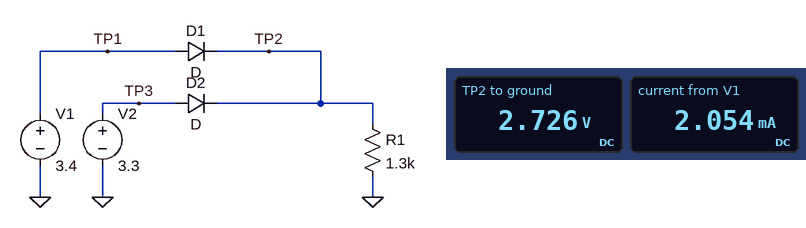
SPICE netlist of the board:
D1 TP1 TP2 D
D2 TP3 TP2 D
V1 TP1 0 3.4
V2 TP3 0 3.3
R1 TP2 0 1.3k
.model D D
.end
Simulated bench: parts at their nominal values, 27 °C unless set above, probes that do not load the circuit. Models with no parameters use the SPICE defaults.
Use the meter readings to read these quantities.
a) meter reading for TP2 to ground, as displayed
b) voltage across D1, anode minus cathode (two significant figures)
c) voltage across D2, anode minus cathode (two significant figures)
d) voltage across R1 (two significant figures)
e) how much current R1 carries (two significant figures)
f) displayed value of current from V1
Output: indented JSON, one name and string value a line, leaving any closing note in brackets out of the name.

{
  "meter reading for TP2 to ground, as displayed": "2.726 V",
  "voltage across D1, anode minus cathode": "670 mV",
  "voltage across D2, anode minus cathode": "570 mV",
  "voltage across R1": "2.7 V",
  "how much current R1 carries": "2.1 mA",
  "displayed value of current from V1": "2.054 mA"
}
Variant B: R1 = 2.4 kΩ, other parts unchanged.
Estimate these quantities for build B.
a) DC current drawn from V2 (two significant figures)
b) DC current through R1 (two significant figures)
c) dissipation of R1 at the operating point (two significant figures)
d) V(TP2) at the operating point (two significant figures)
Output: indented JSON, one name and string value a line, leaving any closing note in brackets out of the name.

{
  "DC current drawn from V2": "23 µA",
  "DC current through R1": "1.1 mA",
  "dissipation of R1 at the operating point": "3.1 mW",
  "V(TP2) at the operating point": "2.7 V"
}
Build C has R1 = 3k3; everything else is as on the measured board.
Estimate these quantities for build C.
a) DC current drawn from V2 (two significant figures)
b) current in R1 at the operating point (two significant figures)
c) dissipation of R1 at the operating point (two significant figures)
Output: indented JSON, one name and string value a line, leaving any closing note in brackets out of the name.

{
  "DC current drawn from V2": "17 µA",
  "current in R1 at the operating point": "830 µA",
  "dissipation of R1 at the operating point": "2.3 mW"
}
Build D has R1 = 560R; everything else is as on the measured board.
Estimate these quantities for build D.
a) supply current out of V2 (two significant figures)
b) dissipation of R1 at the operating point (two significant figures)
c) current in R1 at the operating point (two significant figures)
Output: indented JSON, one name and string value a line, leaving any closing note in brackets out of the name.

{
  "supply current out of V2": "99 µA",
  "dissipation of R1 at the operating point": "13 mW",
  "current in R1 at the operating point": "4.8 mA"
}
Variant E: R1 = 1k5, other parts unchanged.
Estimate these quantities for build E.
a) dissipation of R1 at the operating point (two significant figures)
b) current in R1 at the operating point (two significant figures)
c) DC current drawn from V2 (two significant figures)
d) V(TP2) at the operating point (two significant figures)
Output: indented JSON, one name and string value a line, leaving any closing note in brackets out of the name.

{
  "dissipation of R1 at the operating point": "5.0 mW",
  "current in R1 at the operating point": "1.8 mA",
  "DC current drawn from V2": "37 µA",
  "V(TP2) at the operating point": "2.7 V"
}
